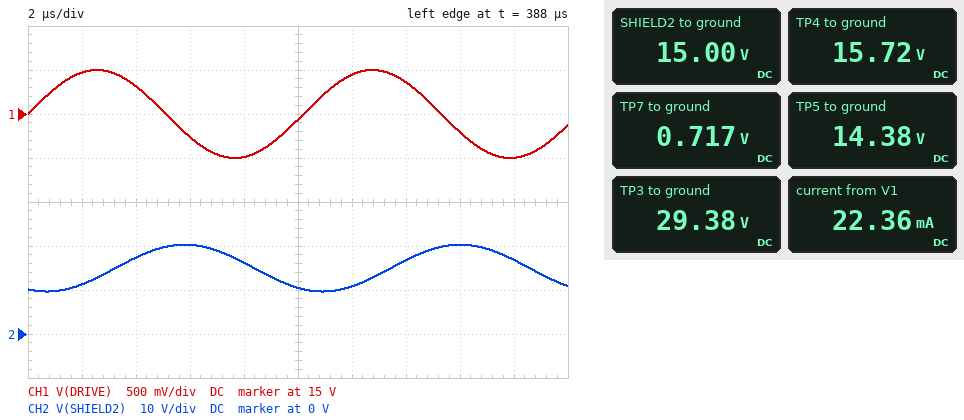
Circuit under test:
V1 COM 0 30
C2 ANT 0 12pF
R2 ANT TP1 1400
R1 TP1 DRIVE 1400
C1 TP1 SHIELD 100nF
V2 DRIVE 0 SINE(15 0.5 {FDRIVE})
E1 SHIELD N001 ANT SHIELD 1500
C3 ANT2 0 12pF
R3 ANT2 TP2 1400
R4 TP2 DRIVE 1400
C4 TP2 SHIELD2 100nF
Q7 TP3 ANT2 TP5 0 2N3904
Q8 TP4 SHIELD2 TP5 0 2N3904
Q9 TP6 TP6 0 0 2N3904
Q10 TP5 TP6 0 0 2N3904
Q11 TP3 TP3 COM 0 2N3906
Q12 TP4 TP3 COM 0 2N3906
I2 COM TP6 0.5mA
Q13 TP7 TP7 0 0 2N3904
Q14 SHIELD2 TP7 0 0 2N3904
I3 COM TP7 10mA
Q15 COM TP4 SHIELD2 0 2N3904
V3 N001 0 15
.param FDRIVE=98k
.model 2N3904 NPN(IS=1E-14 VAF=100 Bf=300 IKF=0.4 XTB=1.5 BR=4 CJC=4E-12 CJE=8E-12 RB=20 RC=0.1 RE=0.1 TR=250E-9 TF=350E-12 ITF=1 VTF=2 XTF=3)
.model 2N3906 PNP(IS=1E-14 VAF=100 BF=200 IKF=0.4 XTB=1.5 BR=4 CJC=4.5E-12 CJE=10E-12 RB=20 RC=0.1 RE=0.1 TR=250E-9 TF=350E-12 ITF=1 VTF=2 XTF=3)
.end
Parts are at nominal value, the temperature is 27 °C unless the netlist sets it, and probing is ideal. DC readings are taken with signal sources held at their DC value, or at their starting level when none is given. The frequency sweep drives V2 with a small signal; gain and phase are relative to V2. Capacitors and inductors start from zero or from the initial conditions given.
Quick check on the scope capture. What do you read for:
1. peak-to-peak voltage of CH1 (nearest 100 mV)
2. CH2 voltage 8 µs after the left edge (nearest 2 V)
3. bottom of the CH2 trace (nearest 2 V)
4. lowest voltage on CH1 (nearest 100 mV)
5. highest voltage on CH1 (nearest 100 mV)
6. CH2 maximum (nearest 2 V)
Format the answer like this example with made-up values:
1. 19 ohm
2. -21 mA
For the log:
1. 1.0 V
2. 16 V
3. 10 V
4. 14.5 V
5. 15.5 V
6. 20 V
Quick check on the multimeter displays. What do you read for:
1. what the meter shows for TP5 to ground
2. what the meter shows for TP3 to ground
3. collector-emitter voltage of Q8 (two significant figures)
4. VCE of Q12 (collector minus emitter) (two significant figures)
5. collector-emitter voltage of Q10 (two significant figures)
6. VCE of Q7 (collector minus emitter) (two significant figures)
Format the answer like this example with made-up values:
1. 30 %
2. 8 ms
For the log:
1. 14.38 V
2. 29.38 V
3. 1.3 V
4. -14 V
5. 14 V
6. 15 V
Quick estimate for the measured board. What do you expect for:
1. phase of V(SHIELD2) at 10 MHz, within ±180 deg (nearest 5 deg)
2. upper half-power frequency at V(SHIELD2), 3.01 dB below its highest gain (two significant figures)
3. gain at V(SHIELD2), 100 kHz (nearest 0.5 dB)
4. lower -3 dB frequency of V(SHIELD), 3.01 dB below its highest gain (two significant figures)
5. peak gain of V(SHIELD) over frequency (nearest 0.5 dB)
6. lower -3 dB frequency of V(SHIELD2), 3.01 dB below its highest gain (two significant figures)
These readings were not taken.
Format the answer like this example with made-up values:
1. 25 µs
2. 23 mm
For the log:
1. 60 deg
2. 100 kHz
3. 18.5 dB
4. 99 kHz
5. 21.5 dB
6. 92 kHz
